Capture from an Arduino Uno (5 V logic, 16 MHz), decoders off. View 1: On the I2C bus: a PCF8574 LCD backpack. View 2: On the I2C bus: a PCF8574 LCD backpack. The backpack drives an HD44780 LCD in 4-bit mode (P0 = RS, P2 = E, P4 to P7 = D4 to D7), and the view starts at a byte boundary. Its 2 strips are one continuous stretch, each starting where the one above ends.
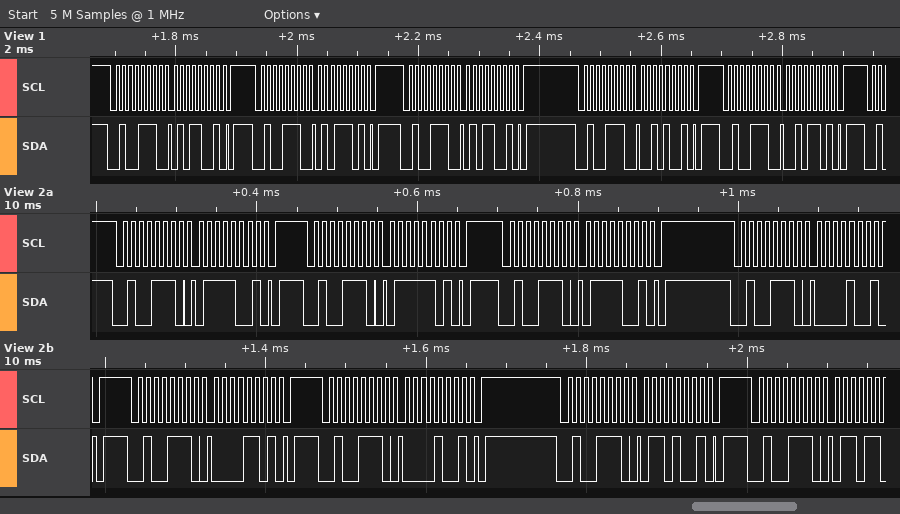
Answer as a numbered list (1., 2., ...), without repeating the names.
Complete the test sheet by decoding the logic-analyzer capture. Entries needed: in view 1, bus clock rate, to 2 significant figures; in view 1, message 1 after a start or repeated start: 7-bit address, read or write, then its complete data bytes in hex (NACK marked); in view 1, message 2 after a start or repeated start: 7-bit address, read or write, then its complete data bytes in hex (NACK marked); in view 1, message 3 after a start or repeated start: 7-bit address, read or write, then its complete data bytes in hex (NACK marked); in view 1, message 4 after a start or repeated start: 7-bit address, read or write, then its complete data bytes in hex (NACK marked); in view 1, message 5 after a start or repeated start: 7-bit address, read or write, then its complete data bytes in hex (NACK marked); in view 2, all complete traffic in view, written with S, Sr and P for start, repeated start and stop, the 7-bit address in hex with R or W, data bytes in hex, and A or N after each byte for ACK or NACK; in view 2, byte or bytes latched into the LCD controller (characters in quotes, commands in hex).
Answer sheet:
1. 100 kHz
2. 0x27 write: 59
3. 0x27 write: 5D
4. 0x27 write: 59
5. 0x27 write: 29
6. 0x27 write: 2D
7. S 27W A 79 A P S 27W A 7D A P S 27W A 79 A P S 27W A 09 A P S 27W A 0D A P S 27W A 09 A P S 27W A 69 A P S 27W A
8. 'p'
